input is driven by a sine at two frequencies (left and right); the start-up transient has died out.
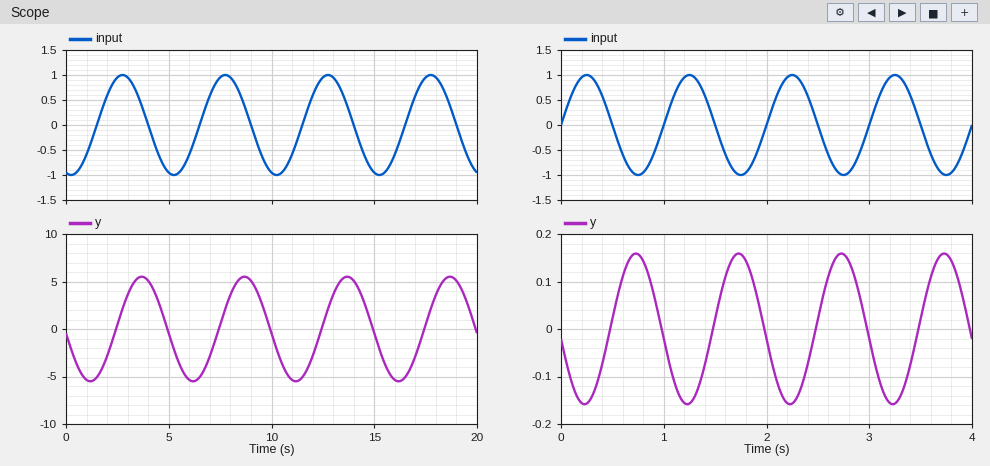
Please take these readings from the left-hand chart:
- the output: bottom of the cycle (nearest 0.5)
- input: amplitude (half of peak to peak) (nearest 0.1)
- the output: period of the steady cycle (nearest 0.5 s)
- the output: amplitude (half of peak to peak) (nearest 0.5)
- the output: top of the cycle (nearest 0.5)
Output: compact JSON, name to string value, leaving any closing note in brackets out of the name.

{"the output: bottom of the cycle": "-5.5", "input: amplitude (half of peak to peak)": "1.0", "the output: period of the steady cycle": "5.0 s", "the output: amplitude (half of peak to peak)": "5.5", "the output: top of the cycle": "5.5"}
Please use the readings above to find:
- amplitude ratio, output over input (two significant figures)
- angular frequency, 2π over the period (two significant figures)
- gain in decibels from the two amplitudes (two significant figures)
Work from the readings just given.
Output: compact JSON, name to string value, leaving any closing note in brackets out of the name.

{"amplitude ratio, output over input": "5.5", "angular frequency, 2π over the period": "1.3 rad/s", "gain in decibels from the two amplitudes": "15 dB"}
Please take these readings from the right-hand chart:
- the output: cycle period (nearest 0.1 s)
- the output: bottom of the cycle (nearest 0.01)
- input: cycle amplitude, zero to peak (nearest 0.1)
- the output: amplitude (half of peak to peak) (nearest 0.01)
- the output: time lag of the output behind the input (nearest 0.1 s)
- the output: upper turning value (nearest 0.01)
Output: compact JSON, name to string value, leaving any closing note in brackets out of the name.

{"the output: cycle period": "1.0 s", "the output: bottom of the cycle": "-0.16", "input: cycle amplitude, zero to peak": "1.0", "the output: amplitude (half of peak to peak)": "0.16", "the output: time lag of the output behind the input": "0.5 s", "the output: upper turning value": "0.16"}
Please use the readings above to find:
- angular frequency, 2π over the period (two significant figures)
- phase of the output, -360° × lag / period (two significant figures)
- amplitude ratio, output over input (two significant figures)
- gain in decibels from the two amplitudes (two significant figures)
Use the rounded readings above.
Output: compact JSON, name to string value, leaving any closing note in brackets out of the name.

{"angular frequency, 2π over the period": "6.3 rad/s", "phase of the output, -360° × lag / period": "-180°", "amplitude ratio, output over input": "0.16", "gain in decibels from the two amplitudes": "-16 dB"}
